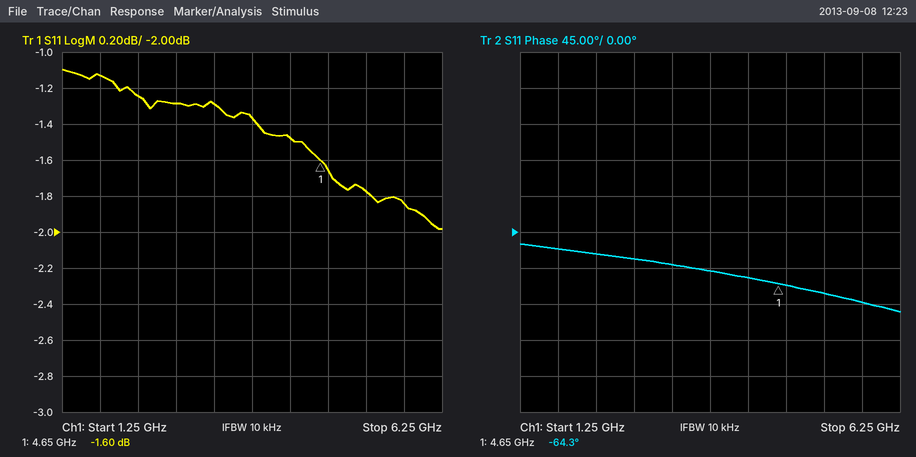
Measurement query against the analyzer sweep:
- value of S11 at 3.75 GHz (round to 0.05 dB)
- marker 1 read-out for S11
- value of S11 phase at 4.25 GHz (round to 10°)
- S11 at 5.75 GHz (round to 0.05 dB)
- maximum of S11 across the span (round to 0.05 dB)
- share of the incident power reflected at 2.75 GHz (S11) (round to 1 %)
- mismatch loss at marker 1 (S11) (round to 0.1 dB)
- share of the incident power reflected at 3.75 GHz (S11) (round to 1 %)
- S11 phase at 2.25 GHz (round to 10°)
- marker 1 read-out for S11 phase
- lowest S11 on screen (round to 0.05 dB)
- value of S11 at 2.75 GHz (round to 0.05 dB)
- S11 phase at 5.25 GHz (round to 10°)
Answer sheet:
-1.35 dB
-1.60 dB
-60°
-1.85 dB
-1.10 dB
74 %
5.1 dB
73 %
-30°
-64.3°
-2.00 dB
-1.30 dB
-80°
